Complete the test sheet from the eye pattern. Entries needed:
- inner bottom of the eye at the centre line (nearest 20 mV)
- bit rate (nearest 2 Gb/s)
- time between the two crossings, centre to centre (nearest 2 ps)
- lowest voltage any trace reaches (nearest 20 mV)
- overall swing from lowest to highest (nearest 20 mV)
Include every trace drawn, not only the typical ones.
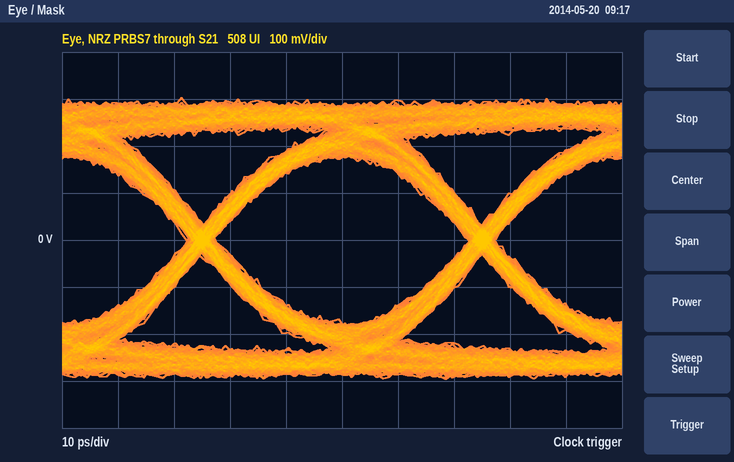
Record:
-180 mV
20 Gb/s
50 ps
-300 mV
600 mV
